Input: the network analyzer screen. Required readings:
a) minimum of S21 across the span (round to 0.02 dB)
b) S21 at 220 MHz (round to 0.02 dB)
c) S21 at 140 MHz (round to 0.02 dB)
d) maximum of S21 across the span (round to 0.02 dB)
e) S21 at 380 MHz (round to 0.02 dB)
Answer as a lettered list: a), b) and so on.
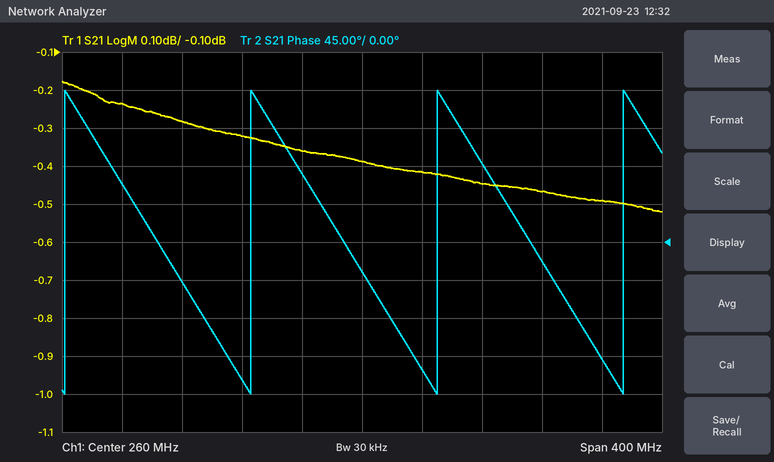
a) -0.52 dB
b) -0.36 dB
c) -0.28 dB
d) -0.18 dB
e) -0.46 dB
